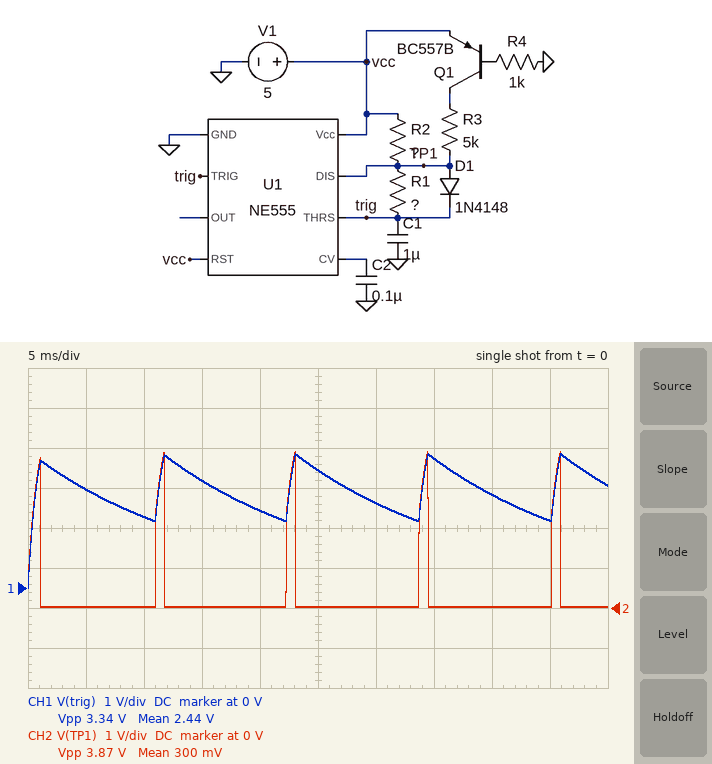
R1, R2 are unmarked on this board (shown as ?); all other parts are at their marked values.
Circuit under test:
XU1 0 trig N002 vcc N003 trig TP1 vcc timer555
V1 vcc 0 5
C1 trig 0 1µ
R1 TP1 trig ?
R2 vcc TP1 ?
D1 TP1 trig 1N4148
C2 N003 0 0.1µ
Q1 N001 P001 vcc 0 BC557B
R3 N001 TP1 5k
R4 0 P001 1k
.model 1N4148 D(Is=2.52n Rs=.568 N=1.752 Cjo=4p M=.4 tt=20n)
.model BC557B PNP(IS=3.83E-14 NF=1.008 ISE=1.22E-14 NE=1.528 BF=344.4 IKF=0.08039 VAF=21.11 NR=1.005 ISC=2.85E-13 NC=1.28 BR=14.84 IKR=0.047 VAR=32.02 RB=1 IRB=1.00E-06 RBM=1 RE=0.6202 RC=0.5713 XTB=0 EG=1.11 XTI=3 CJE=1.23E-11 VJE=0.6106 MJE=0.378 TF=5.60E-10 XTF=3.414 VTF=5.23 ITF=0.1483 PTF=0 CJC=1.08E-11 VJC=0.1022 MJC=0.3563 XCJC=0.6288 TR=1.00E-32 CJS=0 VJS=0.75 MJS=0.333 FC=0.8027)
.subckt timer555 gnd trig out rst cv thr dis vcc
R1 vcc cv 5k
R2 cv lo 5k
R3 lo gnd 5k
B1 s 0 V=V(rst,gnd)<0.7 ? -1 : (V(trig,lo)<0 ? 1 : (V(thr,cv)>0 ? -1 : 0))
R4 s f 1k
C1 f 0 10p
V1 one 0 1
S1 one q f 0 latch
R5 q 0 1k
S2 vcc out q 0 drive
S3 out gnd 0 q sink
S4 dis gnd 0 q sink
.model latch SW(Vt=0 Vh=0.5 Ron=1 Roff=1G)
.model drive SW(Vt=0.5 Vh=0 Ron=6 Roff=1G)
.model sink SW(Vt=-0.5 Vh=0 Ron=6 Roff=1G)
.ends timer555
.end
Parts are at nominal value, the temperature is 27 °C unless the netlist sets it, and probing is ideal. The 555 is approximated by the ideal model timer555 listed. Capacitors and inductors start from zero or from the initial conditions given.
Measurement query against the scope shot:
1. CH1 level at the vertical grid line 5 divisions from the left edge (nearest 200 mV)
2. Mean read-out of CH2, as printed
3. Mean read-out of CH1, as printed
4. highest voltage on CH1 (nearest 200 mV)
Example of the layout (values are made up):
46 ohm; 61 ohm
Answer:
3.0 V; 300 mV; 2.44 V; 3.4 V
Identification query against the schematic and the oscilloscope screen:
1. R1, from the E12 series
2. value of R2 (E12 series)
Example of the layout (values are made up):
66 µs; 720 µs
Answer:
15 kΩ; 1 kΩ
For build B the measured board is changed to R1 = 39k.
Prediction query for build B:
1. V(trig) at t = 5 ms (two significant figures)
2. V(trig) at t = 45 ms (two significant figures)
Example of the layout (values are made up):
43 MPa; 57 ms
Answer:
2.9 V; 2.2 V
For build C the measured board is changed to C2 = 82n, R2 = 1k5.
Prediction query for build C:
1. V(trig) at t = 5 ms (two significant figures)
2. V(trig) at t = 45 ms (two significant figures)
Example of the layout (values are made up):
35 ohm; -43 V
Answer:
2.7 V; 1.9 V
